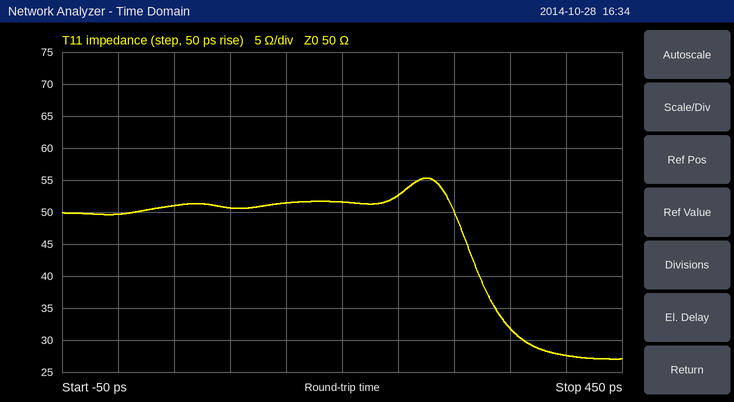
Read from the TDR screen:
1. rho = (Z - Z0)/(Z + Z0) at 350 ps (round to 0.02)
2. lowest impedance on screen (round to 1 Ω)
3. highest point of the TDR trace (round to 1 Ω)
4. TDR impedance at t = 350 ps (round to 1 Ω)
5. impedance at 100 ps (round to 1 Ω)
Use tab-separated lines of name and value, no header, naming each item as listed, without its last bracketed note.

rho = (Z - Z0)/(Z + Z0) at 350 ps	-0.22
lowest impedance on screen	27 Ω
highest point of the TDR trace	55 Ω
TDR impedance at t = 350 ps	32 Ω
impedance at 100 ps	51 Ω
